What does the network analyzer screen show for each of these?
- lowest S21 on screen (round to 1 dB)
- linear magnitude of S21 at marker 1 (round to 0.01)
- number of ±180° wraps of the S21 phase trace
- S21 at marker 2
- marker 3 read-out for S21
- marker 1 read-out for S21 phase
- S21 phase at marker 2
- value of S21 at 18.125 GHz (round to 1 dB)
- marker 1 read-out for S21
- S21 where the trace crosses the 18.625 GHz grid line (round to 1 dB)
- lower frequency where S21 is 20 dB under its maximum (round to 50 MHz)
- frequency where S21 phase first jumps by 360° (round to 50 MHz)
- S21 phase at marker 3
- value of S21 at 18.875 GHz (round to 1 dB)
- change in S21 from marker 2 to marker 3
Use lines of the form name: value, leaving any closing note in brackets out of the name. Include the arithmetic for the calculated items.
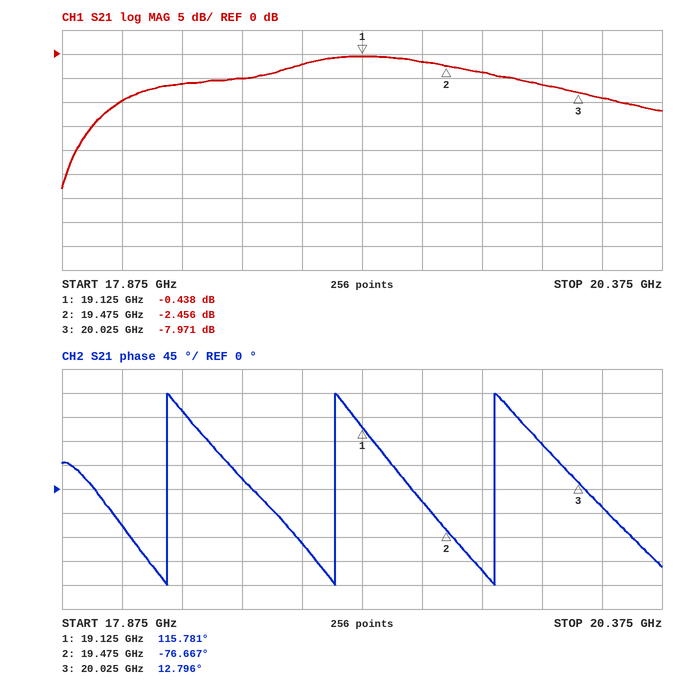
lowest S21 on screen: -28 dB
linear magnitude of S21 at marker 1: 10^(-0.438/20) ≈ 0.95
number of ±180° wraps of the S21 phase trace: 3
S21 at marker 2: -2.456 dB
marker 3 read-out for S21: -7.971 dB
marker 1 read-out for S21 phase: 115.781°
S21 phase at marker 2: -76.667°
value of S21 at 18.125 GHz: -10 dB
marker 1 read-out for S21: -0.438 dB
S21 where the trace crosses the 18.625 GHz grid line: -5 dB
lower frequency where S21 is 20 dB under its maximum: 17.95 GHz
frequency where S21 phase first jumps by 360°: 18.30 GHz
S21 phase at marker 3: 12.796°
value of S21 at 18.875 GHz: -2 dB
change in S21 from marker 2 to marker 3: -7.971 − (-2.456) = -5.515 dB
